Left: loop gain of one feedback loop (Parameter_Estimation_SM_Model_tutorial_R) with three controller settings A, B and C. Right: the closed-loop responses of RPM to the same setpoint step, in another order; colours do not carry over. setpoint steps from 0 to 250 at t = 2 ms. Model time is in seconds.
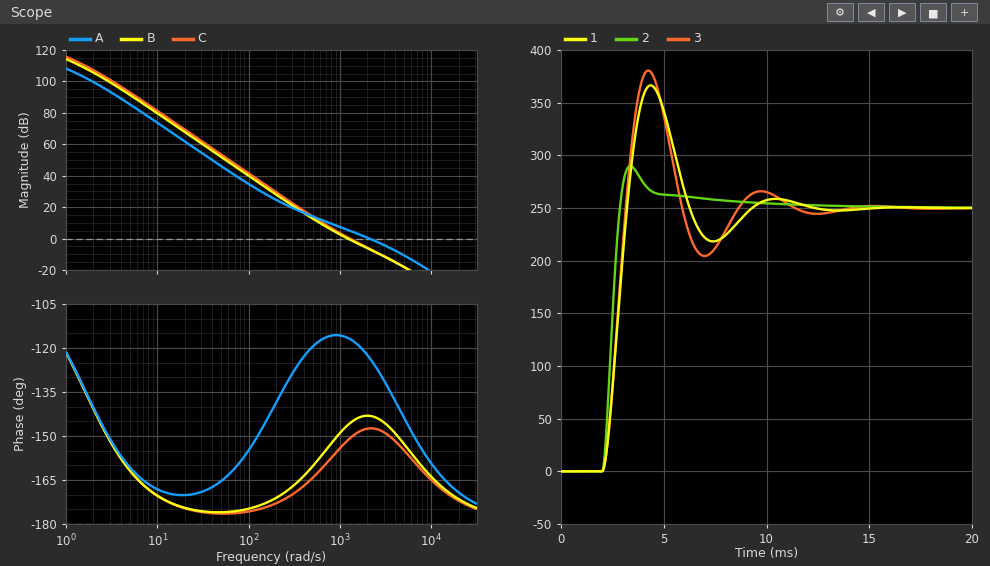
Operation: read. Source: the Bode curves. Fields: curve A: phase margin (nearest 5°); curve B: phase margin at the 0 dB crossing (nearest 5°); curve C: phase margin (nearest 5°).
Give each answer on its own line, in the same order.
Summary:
55°
35°
30°
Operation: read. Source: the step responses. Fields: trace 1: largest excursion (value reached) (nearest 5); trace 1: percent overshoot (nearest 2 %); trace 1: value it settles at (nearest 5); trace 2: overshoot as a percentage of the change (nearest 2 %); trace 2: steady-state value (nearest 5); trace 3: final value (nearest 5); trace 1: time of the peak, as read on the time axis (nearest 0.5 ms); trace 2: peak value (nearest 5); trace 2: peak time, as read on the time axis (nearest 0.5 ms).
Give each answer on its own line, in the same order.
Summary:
365
46 %
250
16 %
250
250
4.5 ms
290
3.5 ms
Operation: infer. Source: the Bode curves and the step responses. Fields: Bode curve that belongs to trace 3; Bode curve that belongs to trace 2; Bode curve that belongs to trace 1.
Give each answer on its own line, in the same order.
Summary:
C
A
B
